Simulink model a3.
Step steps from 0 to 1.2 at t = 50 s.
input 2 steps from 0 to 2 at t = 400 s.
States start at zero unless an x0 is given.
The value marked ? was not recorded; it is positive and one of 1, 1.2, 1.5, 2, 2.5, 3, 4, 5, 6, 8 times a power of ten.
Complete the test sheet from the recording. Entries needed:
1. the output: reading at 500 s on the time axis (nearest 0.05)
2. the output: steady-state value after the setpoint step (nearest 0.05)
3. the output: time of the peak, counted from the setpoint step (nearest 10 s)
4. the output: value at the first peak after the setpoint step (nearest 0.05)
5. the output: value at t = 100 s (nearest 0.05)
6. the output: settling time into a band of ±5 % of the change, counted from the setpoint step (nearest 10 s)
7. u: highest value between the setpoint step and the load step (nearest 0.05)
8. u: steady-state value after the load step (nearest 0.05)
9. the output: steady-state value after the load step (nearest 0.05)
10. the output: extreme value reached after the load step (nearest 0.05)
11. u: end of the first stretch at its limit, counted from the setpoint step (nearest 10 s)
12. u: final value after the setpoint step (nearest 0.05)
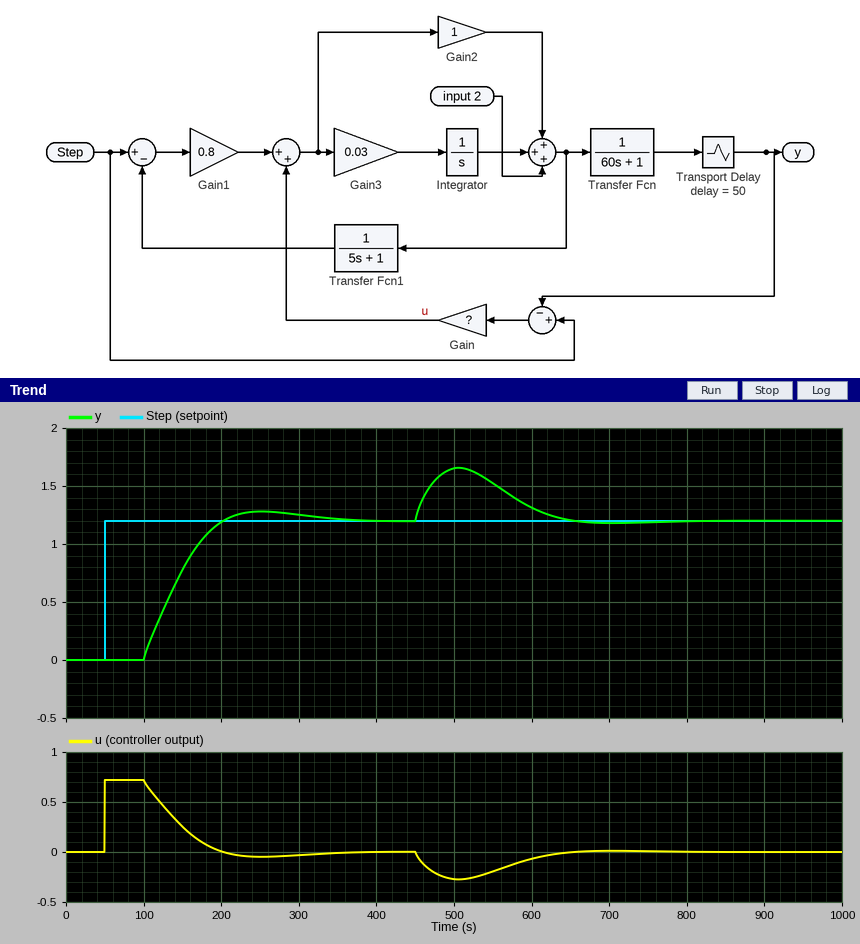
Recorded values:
1.65
1.20
200 s
1.30
0.00
240 s
0.70
0.00
1.20
1.65
50 s
0.00
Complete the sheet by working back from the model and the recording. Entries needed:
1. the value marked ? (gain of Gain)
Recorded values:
0.6
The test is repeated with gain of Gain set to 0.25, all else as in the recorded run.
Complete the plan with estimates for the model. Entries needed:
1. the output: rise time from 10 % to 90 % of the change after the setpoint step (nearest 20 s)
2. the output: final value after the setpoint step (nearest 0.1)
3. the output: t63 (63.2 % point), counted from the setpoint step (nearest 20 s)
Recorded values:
120 s
1.2
120 s
